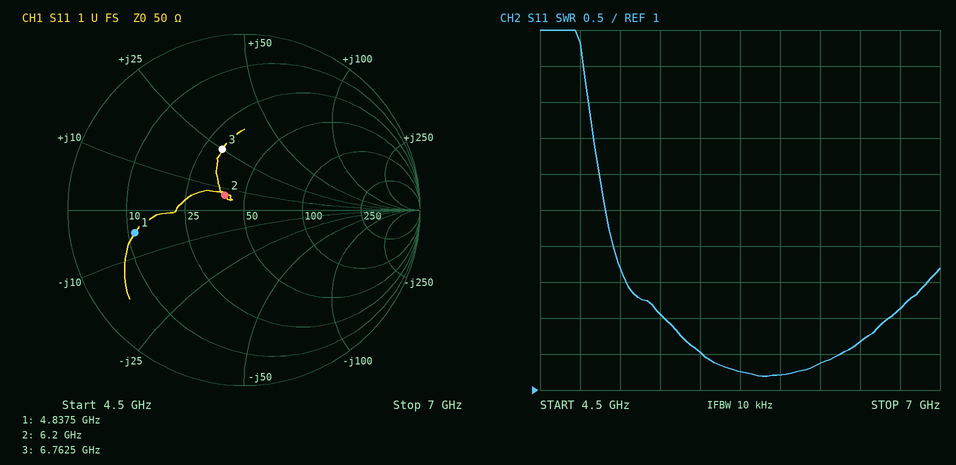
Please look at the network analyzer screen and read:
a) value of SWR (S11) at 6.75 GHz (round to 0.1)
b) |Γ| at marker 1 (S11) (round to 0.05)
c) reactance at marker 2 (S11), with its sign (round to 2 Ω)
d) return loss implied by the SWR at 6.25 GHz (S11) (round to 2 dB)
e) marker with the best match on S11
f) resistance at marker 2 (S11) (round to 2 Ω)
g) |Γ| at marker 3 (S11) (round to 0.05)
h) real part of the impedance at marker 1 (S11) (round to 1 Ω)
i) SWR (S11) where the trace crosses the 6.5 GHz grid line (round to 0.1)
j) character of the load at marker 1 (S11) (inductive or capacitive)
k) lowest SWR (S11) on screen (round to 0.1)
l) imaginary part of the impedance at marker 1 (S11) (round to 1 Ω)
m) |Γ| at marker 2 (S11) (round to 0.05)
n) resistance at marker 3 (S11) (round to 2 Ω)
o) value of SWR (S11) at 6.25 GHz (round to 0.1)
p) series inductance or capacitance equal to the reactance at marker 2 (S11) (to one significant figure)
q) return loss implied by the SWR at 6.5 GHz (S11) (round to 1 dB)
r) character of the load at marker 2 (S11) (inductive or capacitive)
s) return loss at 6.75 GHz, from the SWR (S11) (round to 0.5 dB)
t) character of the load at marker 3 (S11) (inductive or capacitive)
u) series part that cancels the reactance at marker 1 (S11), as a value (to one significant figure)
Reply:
2.1
0.65
+6 Ω
16 dB
marker 2
40 Ω
0.35
11 Ω
1.7
capacitive
1.2
-5 Ω
0.15
32 Ω
1.4
200 pH
12 dB
inductive
9.0 dB
inductive
200 pH
